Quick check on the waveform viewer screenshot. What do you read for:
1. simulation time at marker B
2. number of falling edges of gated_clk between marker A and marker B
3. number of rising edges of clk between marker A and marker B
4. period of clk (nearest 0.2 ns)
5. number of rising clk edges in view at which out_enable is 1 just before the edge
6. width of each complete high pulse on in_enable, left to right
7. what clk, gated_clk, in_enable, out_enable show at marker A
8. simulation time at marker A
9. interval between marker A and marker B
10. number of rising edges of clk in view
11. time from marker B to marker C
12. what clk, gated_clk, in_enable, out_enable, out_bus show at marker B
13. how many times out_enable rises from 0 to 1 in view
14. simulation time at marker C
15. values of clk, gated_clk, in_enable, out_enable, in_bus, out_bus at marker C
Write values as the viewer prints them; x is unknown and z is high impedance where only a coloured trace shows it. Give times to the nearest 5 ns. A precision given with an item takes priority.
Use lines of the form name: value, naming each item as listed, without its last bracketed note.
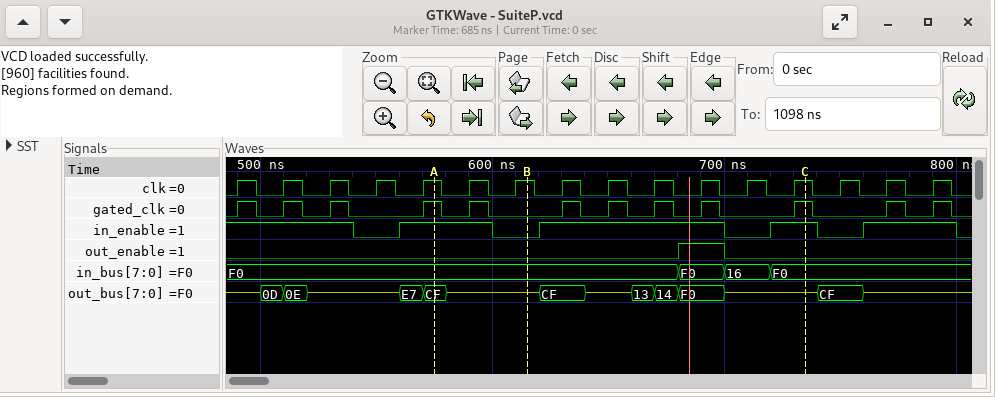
simulation time at marker B: 615 ns
number of falling edges of gated_clk between marker A and marker B: 2
number of rising edges of clk between marker A and marker B: 2
period of clk: 20 ns
number of rising clk edges in view at which out_enable is 1 just before the edge: 1
width of each complete high pulse on in_enable, left to right: 40 ns, 80 ns, 20 ns, 40 ns
what clk, gated_clk, in_enable, out_enable show at marker A: clk=1, gated_clk=1, in_enable=1, out_enable=0
simulation time at marker A: 575 ns
interval between marker A and marker B: 40 ns
number of rising edges of clk in view: 16
time from marker B to marker C: 120 ns
what clk, gated_clk, in_enable, out_enable, out_bus show at marker B: clk=1, gated_clk=0, in_enable=0, out_enable=0, out_bus=z
how many times out_enable rises from 0 to 1 in view: 1
simulation time at marker C: 735 ns
values of clk, gated_clk, in_enable, out_enable, in_bus, out_bus at marker C: clk=1, gated_clk=1, in_enable=1, out_enable=0, in_bus=F0, out_bus=z
